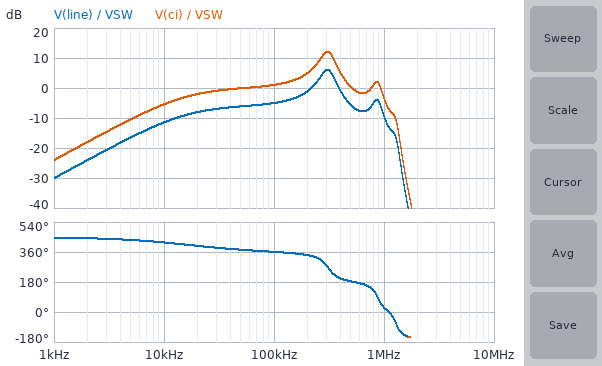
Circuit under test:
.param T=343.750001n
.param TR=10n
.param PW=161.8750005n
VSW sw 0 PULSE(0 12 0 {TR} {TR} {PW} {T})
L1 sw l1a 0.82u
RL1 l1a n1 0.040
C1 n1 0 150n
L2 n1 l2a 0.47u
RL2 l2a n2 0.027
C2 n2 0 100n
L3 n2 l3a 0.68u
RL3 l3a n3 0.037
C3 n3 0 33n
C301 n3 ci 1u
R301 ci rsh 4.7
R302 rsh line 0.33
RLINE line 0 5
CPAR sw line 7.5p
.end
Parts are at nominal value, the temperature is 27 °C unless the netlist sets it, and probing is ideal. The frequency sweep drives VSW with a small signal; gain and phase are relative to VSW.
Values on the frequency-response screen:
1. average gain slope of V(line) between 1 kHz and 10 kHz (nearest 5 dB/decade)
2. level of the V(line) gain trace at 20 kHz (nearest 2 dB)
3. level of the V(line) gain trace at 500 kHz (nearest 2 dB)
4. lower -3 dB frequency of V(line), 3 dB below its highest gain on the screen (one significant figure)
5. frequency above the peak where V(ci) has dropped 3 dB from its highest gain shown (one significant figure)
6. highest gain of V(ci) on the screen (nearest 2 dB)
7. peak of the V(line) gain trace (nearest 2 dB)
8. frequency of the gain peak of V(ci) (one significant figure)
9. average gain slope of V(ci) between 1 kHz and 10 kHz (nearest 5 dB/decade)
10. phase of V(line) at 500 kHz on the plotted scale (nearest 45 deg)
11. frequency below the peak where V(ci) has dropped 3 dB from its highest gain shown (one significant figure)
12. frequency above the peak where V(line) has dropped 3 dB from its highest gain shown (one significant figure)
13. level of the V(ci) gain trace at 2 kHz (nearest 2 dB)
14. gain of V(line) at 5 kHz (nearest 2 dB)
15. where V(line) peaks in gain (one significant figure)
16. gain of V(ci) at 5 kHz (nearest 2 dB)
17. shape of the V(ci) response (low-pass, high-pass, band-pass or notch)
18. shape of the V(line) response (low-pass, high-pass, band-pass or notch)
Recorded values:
20 dB/decade
-8 dB
-6 dB
300 kHz
400 kHz
12 dB
6 dB
300 kHz
20 dB/decade
180 deg
300 kHz
400 kHz
-18 dB
-16 dB
300 kHz
-10 dB
band-pass
band-pass
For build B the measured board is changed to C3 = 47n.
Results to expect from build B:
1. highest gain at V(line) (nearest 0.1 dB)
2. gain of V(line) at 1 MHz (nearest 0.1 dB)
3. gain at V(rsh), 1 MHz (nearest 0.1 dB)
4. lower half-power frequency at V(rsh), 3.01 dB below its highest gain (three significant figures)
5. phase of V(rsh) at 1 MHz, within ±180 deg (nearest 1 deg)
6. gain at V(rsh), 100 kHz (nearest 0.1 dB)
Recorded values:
6.0 dB
-11.9 dB
-11.3 dB
247 kHz
20 deg
-4.4 dB
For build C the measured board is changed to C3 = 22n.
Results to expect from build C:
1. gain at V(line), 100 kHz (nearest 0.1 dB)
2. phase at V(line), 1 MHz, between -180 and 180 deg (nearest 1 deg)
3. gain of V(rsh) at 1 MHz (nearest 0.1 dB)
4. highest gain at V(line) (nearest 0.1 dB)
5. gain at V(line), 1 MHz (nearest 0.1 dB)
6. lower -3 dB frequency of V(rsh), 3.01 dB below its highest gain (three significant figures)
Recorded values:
-5.1 dB
36 deg
-6.5 dB
6.2 dB
-7.0 dB
267 kHz
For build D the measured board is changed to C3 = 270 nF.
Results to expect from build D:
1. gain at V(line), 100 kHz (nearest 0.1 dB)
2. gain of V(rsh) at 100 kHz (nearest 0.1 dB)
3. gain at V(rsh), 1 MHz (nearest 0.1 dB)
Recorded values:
-3.1 dB
-2.6 dB
-25.7 dB
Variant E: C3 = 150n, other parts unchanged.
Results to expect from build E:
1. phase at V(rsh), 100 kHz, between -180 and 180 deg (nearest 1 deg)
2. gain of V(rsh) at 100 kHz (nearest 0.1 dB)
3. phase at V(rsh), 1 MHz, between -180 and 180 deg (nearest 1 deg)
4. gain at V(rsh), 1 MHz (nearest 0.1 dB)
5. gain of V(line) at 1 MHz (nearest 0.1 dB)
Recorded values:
-1 deg
-3.6 dB
6 deg
-20.7 dB
-21.2 dB
